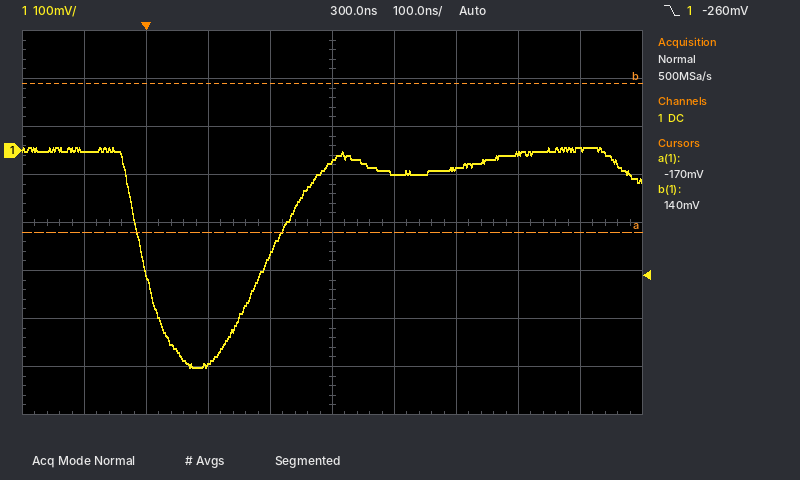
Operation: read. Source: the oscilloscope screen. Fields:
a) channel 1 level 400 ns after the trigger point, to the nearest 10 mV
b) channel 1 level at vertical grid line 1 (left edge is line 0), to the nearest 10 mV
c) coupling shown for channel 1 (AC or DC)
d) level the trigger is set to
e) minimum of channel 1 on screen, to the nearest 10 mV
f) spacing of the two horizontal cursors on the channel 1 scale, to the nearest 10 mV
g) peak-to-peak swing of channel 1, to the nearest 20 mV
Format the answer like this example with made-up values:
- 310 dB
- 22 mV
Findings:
- -50 mV
- 0 mV
- DC
- -260 mV
- -450 mV
- 310 mV
- 460 mV
